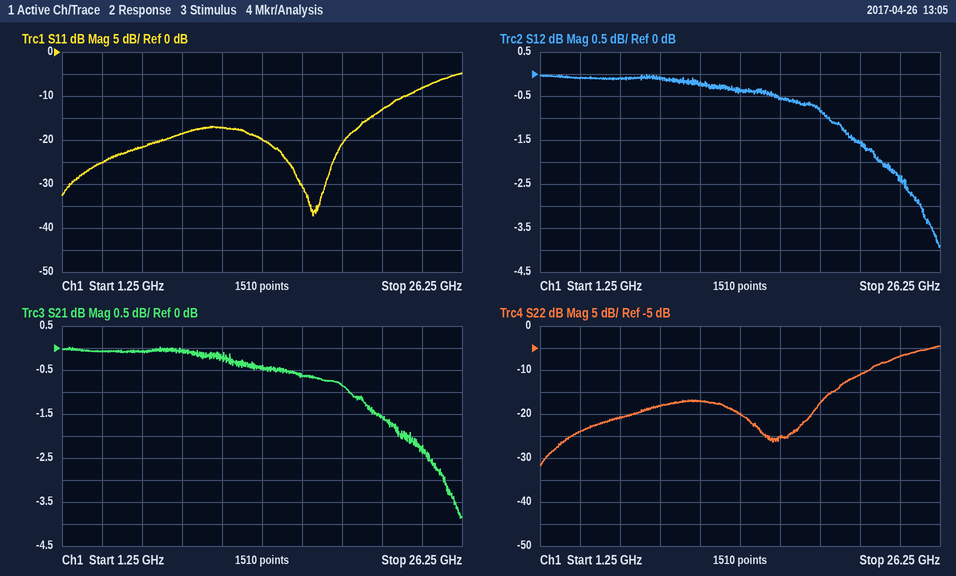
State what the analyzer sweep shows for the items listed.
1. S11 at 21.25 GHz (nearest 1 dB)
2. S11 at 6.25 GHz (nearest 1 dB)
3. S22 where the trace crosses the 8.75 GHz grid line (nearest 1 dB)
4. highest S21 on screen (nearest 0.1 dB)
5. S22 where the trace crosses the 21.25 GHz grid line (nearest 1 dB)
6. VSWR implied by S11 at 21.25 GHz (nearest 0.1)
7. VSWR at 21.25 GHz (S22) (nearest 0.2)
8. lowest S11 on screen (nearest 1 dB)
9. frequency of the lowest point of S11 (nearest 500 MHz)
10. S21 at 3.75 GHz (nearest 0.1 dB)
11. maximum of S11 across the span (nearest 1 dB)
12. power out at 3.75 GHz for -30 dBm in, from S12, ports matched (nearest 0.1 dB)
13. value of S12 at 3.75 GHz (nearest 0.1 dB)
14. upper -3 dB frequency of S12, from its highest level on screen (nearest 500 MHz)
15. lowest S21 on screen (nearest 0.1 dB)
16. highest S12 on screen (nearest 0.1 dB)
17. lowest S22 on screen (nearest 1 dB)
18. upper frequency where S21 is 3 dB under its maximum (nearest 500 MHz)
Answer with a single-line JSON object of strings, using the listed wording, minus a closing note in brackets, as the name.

{"S11 at 21.25 GHz": "-13 dB", "S11 at 6.25 GHz": "-22 dB", "S22 where the trace crosses the 8.75 GHz grid line": "-18 dB", "highest S21 on screen": "0.0 dB", "S22 where the trace crosses the 21.25 GHz grid line": "-11 dB", "VSWR implied by S11 at 21.25 GHz": "1.6", "VSWR at 21.25 GHz (S22)": "1.8", "lowest S11 on screen": "-37 dB", "frequency of the lowest point of S11": "17.0 GHz", "S21 at 3.75 GHz": "-0.1 dB", "maximum of S11 across the span": "-5 dB", "power out at 3.75 GHz for -30 dBm in, from S12, ports matched": "-30.1 dBm", "value of S12 at 3.75 GHz": "-0.1 dB", "upper -3 dB frequency of S12, from its highest level on screen": "25.0 GHz", "lowest S21 on screen": "-3.9 dB", "highest S12 on screen": "0.0 dB", "lowest S22 on screen": "-32 dB", "upper frequency where S21 is 3 dB under its maximum": "25.0 GHz"}
